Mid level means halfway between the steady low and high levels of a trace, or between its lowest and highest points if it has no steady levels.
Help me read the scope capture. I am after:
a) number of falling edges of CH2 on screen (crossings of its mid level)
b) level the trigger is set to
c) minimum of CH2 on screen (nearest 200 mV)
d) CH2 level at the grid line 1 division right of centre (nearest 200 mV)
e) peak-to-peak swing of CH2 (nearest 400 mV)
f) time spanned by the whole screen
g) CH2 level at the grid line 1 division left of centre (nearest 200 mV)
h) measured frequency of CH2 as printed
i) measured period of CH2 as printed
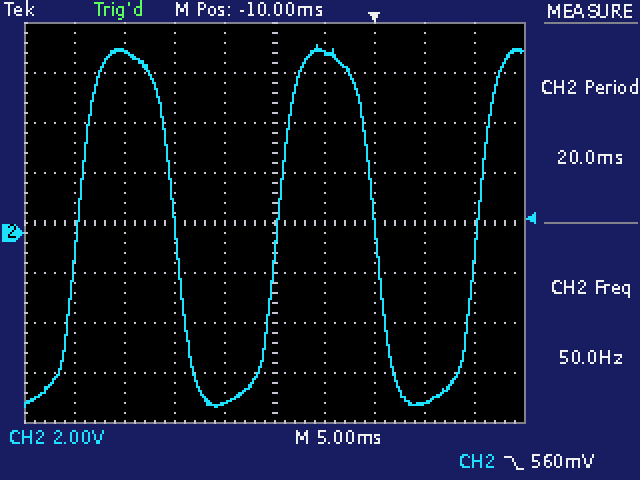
2
560 mV
-7.0 V
7.2 V
14.4 V
50 ms
-6.8 V
50.0 Hz
20.0 ms
